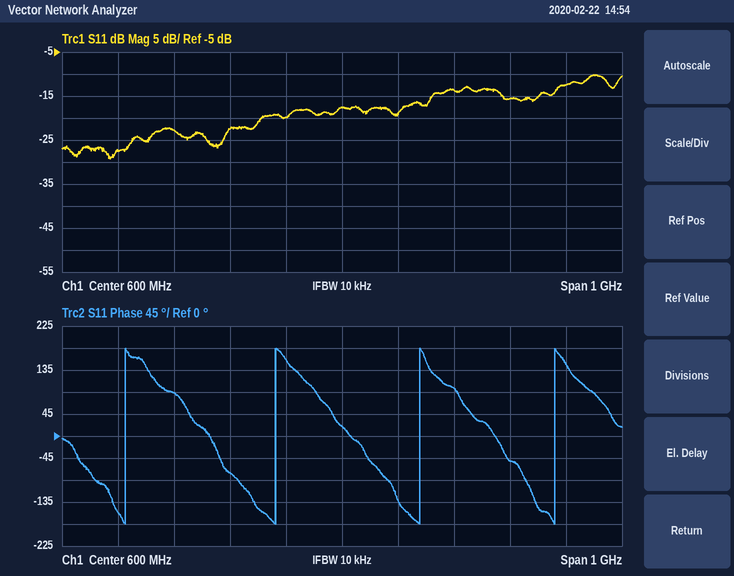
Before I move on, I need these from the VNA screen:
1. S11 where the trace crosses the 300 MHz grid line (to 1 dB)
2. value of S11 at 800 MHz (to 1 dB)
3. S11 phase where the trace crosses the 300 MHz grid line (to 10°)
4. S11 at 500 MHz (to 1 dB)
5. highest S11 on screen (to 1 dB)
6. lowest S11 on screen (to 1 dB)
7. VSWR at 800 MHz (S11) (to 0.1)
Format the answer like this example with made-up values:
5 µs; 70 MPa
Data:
-23 dB; -14 dB; 90°; -20 dB; -10 dB; -29 dB; 1.5
